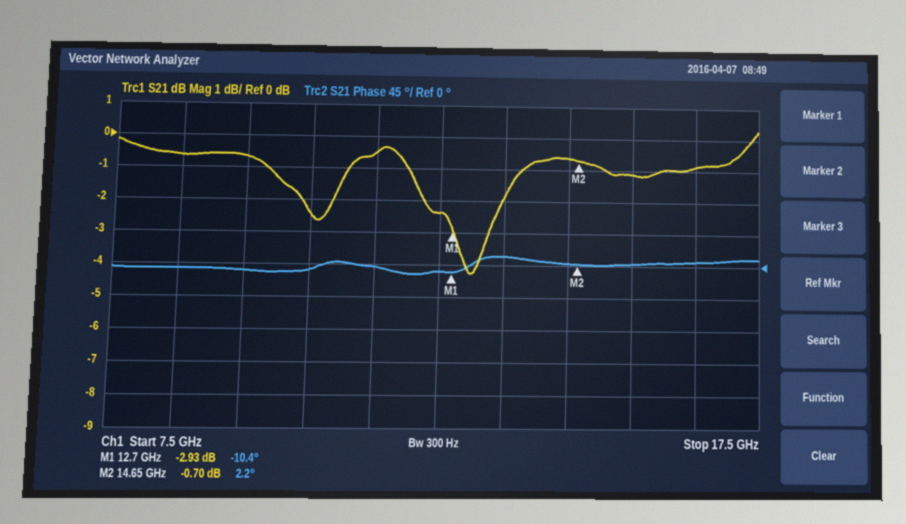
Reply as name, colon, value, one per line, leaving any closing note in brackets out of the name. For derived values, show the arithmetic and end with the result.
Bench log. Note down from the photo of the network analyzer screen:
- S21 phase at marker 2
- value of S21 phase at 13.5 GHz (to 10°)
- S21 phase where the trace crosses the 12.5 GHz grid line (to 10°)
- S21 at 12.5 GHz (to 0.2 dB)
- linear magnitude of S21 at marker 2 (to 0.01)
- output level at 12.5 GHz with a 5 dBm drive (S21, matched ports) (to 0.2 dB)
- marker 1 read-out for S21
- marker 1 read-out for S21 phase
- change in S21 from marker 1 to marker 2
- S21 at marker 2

S21 phase at marker 2: 2.2°
value of S21 phase at 13.5 GHz: 10°
S21 phase where the trace crosses the 12.5 GHz grid line: -10°
S21 at 12.5 GHz: -2.4 dB
linear magnitude of S21 at marker 2: 10^(-0.7/20) ≈ 0.92
output level at 12.5 GHz with a 5 dBm drive (S21, matched ports): 5 dBm + (-2.4 dB) = 2.6 dBm
marker 1 read-out for S21: -2.93 dB
marker 1 read-out for S21 phase: -10.4°
change in S21 from marker 1 to marker 2: -0.7 − (-2.93) = 2.23 dB
S21 at marker 2: -0.70 dB
